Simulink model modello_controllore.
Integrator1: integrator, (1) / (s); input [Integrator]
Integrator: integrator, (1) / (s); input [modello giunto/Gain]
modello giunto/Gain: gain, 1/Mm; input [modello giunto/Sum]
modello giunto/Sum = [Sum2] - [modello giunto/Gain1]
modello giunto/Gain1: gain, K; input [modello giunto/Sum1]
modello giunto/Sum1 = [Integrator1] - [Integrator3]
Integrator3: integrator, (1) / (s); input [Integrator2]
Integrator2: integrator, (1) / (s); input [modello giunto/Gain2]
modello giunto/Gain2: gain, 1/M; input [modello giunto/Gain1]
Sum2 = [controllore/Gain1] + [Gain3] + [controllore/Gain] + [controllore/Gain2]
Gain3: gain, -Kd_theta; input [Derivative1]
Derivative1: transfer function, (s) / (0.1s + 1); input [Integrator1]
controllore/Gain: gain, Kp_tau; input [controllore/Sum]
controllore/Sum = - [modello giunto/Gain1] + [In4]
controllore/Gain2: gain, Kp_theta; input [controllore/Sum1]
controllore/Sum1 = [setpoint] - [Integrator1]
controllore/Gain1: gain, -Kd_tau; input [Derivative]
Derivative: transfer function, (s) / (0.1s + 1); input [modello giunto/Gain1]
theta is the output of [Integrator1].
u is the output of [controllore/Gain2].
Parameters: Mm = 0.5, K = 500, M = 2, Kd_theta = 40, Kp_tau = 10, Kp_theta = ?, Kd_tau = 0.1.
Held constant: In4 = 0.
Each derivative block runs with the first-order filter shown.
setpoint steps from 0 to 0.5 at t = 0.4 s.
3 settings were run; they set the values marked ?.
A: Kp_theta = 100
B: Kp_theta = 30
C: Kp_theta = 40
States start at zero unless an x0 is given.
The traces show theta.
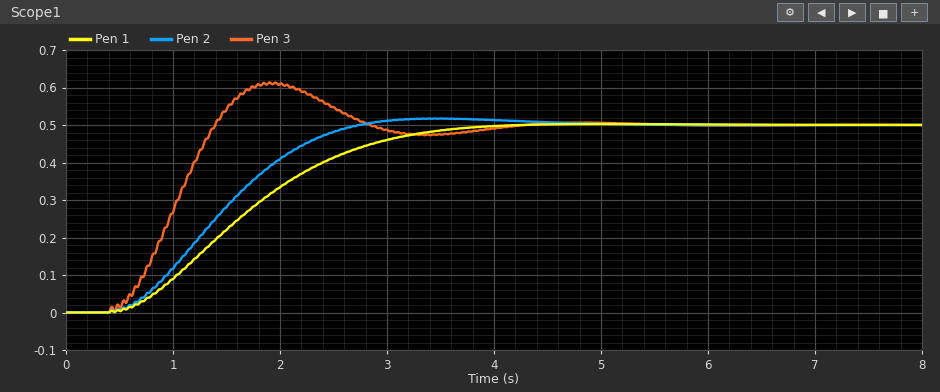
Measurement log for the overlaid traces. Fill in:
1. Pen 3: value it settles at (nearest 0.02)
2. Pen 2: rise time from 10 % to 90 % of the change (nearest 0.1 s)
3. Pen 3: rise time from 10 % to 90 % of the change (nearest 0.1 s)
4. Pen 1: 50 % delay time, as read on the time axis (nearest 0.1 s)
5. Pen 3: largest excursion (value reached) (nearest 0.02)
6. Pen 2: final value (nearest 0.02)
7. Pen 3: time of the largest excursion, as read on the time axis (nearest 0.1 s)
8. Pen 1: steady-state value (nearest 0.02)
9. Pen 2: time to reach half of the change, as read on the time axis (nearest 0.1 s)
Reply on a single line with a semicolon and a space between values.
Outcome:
0.50; 1.5 s; 0.7 s; 1.6 s; 0.62; 0.50; 1.9 s; 0.50; 1.4 s
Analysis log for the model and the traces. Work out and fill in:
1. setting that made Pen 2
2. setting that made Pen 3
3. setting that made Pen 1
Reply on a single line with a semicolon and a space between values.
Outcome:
C; A; B
